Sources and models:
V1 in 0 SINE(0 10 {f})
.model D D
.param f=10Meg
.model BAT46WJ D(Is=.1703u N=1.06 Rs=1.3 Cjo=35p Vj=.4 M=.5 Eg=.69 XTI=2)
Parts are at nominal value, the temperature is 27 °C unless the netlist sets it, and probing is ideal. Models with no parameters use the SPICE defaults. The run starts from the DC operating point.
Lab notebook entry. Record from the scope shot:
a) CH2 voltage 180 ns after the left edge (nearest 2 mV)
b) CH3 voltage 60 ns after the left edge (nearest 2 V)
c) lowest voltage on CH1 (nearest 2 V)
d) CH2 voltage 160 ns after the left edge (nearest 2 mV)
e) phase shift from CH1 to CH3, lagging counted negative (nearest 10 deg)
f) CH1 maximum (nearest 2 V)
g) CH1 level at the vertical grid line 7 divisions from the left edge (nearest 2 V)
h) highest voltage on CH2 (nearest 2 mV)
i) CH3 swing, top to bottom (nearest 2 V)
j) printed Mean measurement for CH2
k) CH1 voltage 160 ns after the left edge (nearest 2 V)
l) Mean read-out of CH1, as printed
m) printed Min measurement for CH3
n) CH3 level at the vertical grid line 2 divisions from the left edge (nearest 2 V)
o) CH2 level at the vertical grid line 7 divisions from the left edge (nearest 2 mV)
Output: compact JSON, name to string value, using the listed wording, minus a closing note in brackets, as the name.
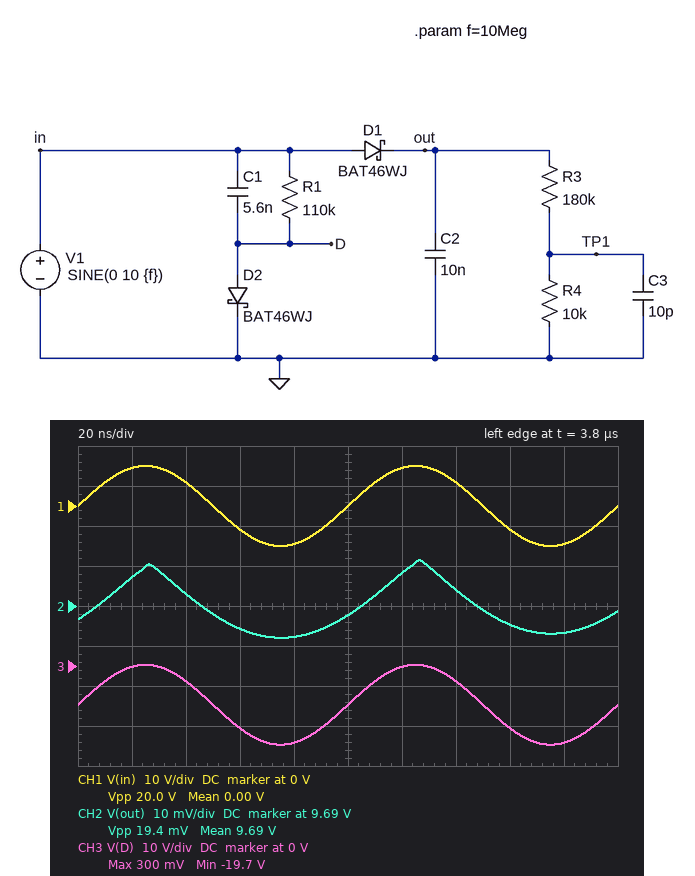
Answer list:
{"CH2 voltage 180 ns after the left edge": "9.684 V", "CH3 voltage 60 ns after the left edge": "-16 V", "lowest voltage on CH1": "-10 V", "CH2 voltage 160 ns after the left edge": "9.686 V", "phase shift from CH1 to CH3, lagging counted negative": "0 deg", "CH1 maximum": "10 V", "CH1 level at the vertical grid line 7 divisions from the left edge": "6 V", "highest voltage on CH2": "9.702 V", "CH3 swing, top to bottom": "20 V", "printed Mean measurement for CH2": "9.69 V", "CH1 voltage 160 ns after the left edge": "-6 V", "Mean read-out of CH1, as printed": "0.00 V", "printed Min measurement for CH3": "-19.7 V", "CH3 level at the vertical grid line 2 divisions from the left edge": "-4 V", "CH2 level at the vertical grid line 7 divisions from the left edge": "9.694 V"}
